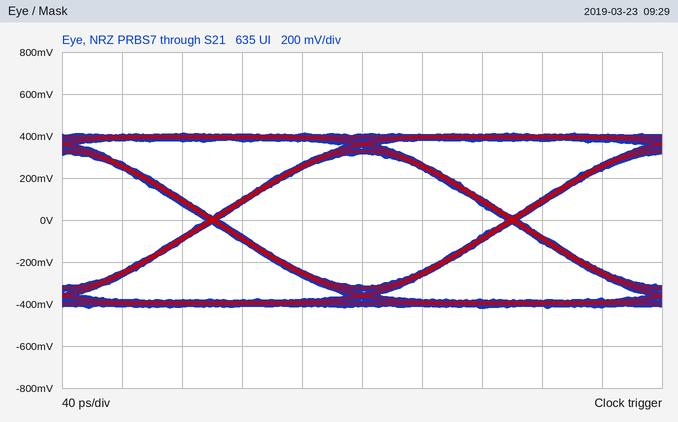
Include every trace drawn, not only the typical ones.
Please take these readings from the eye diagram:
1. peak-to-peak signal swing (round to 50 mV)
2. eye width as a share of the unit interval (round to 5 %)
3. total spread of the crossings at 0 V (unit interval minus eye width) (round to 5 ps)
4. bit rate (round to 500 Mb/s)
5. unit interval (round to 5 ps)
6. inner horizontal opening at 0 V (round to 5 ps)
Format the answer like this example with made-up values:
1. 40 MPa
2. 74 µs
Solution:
1. 850 mV
2. 95 %
3. 10 ps
4. 5.0 Gb/s
5. 200 ps
6. 190 ps
